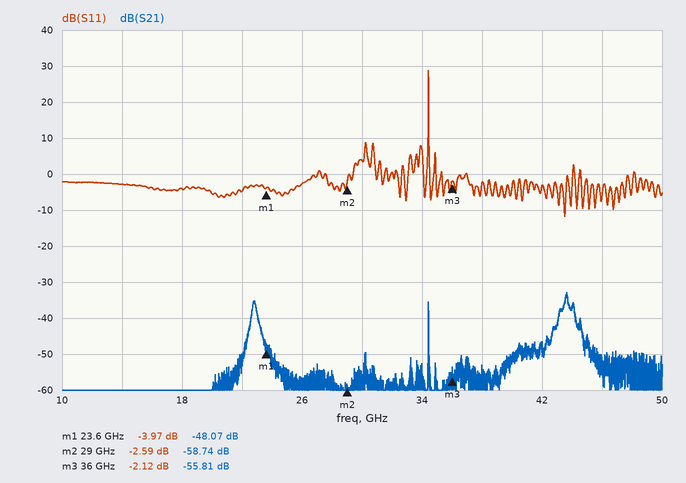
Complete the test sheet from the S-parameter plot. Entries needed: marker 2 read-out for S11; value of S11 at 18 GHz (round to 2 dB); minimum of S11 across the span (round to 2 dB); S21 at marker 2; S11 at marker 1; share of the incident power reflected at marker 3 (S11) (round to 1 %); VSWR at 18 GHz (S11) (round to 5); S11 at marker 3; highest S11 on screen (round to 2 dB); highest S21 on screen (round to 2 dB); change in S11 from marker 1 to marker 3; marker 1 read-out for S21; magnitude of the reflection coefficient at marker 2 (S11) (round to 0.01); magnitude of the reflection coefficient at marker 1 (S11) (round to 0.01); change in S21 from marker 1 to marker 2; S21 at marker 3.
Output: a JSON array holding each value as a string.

["-2.59 dB", "-4 dB", "-12 dB", "-58.74 dB", "-3.97 dB", "61 %", "5", "-2.12 dB", "28 dB", "-32 dB", "1.85 dB", "-48.07 dB", "0.74", "0.63", "-10.67 dB", "-55.81 dB"]
